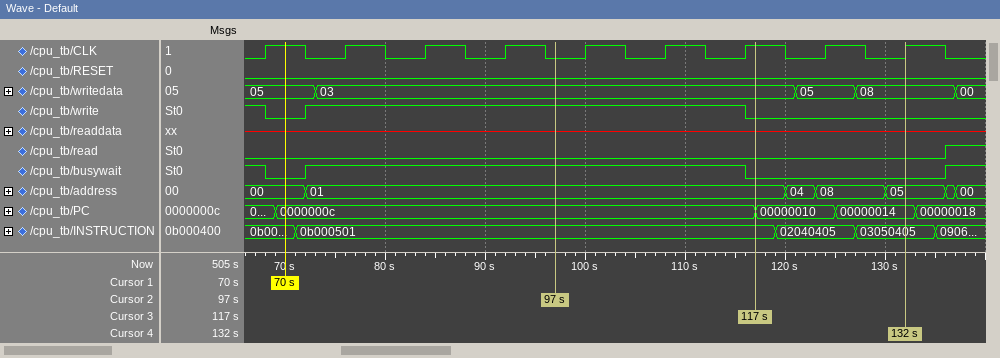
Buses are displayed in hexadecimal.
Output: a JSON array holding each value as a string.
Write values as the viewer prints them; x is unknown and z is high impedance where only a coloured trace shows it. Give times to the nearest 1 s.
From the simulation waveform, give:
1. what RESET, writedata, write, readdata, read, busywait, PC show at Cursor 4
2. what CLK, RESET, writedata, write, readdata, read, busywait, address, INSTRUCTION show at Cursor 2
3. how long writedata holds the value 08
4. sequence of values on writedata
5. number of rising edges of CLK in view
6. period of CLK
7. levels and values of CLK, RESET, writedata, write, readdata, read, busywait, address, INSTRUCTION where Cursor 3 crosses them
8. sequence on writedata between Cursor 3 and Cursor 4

["RESET=0, writedata=08, write=0, readdata=x, read=0, busywait=0, PC=00000014", "CLK=0, RESET=0, writedata=03, write=1, readdata=x, read=0, busywait=1, address=01, INSTRUCTION=0b000501", "10 s", "05, 03, 05, 08, 00", "9", "8 s", "CLK=1, RESET=0, writedata=03, write=0, readdata=x, read=0, busywait=0, address=01, INSTRUCTION=0b000501", "03, 05, 08"]
